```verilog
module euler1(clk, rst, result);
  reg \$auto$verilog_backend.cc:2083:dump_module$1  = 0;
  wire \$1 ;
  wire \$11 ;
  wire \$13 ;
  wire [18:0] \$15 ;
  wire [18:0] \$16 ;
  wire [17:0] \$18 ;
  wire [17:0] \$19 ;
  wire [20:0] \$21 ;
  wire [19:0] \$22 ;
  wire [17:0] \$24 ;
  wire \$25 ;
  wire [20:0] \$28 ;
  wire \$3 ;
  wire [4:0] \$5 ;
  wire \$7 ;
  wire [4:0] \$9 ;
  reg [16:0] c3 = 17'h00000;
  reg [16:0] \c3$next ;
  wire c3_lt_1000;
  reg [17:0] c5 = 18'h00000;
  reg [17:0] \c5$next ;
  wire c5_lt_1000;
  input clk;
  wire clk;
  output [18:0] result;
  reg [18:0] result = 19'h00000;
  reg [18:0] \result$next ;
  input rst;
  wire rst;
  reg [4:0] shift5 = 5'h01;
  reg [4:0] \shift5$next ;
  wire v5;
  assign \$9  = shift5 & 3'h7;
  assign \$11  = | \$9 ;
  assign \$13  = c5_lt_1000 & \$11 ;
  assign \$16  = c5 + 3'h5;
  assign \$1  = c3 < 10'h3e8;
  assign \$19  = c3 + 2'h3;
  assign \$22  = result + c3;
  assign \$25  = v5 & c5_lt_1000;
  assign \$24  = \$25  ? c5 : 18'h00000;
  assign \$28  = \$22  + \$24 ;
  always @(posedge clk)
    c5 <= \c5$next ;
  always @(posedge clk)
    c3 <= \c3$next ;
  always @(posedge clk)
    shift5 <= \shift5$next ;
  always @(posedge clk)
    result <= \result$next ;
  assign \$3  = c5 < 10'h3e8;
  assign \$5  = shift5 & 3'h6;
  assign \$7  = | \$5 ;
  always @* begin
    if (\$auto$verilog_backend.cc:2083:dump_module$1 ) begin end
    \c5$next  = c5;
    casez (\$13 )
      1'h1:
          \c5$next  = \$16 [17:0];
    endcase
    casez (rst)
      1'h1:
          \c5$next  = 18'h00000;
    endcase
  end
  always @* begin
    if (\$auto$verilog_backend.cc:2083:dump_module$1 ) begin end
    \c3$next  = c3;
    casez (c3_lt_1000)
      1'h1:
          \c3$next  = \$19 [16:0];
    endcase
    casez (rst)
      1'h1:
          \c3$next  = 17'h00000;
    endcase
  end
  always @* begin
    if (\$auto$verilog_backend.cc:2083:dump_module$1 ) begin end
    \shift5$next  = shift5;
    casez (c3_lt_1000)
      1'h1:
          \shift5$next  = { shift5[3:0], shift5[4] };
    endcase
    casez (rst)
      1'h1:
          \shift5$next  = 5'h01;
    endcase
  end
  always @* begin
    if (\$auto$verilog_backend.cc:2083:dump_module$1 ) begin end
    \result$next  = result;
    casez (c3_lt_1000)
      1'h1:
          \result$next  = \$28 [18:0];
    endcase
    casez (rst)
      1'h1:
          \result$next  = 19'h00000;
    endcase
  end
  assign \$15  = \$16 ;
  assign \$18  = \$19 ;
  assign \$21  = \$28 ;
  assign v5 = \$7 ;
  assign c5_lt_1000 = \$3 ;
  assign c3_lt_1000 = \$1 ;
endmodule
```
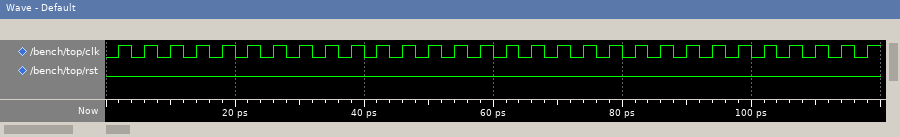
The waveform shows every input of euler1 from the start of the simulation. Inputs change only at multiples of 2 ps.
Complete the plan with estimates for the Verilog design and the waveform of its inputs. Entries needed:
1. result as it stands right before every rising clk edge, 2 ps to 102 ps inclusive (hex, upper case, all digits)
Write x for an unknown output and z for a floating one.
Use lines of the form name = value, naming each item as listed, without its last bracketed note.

result as it stands right before every rising clk edge, 2 ps to 102 ps inclusive = 00000, 00000, 00008, 00018, 00021, 0002D, 0003C, 00062, 00090, 000A8, 000C3, 000E1, 00125, 00171, 00198, 001C2, 001EF, 00251, 002BB, 002F1, 0032A, 00366, 003E6, 0046E, 004B3, 004FB
